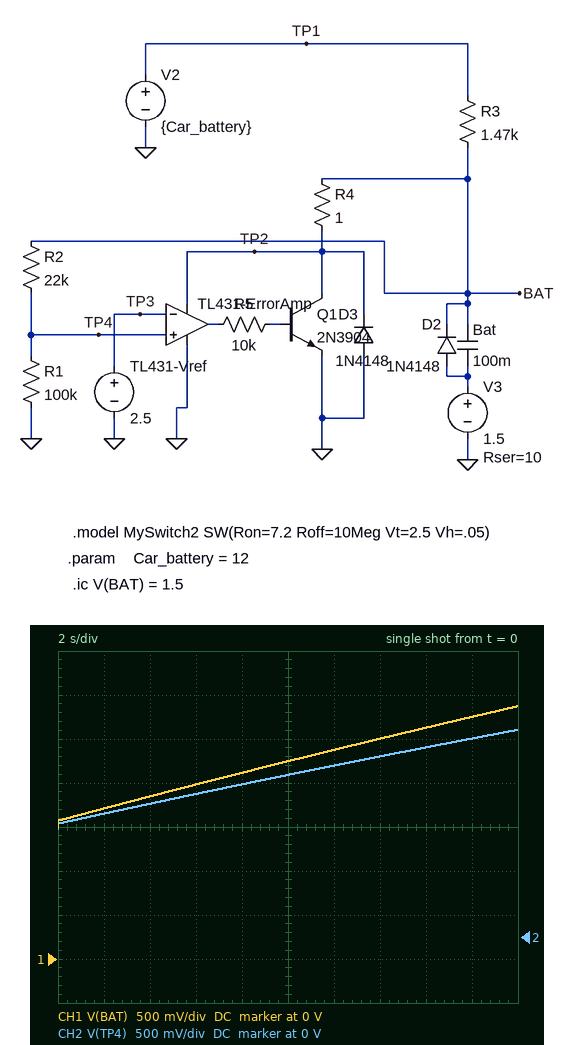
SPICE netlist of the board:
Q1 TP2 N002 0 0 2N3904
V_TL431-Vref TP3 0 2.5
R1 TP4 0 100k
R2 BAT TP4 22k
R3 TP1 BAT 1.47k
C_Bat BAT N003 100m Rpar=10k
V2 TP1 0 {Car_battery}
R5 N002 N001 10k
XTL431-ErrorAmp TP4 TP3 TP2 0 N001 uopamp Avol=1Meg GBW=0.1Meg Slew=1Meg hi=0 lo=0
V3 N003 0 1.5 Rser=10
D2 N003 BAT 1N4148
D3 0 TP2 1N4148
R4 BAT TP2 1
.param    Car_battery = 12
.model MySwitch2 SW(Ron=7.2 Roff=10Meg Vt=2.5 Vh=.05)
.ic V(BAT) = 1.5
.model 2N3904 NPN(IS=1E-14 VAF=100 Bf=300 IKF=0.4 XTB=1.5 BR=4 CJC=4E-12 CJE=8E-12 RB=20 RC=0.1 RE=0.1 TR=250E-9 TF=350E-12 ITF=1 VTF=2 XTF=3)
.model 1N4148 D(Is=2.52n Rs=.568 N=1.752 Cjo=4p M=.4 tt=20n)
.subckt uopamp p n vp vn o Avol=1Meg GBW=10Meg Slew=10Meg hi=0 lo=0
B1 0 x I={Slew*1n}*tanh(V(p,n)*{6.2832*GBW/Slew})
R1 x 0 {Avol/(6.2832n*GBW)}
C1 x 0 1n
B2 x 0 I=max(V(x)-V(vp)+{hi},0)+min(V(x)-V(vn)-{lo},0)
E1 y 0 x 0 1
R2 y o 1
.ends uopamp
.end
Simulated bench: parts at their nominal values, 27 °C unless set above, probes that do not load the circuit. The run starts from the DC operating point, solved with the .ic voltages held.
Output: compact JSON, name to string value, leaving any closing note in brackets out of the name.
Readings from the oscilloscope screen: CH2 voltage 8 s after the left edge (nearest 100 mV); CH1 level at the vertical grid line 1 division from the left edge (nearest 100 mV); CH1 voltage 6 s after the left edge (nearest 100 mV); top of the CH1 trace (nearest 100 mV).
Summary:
{"CH2 voltage 8 s after the left edge": "1.7 V", "CH1 level at the vertical grid line 1 division from the left edge": "1.7 V", "CH1 voltage 6 s after the left edge": "2.0 V", "top of the CH1 trace": "2.9 V"}
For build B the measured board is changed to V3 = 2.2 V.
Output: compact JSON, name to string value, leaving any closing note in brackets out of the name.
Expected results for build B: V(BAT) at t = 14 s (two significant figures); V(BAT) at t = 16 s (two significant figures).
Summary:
{"V(BAT) at t = 14 s": "2.6 V", "V(BAT) at t = 16 s": "2.7 V"}
